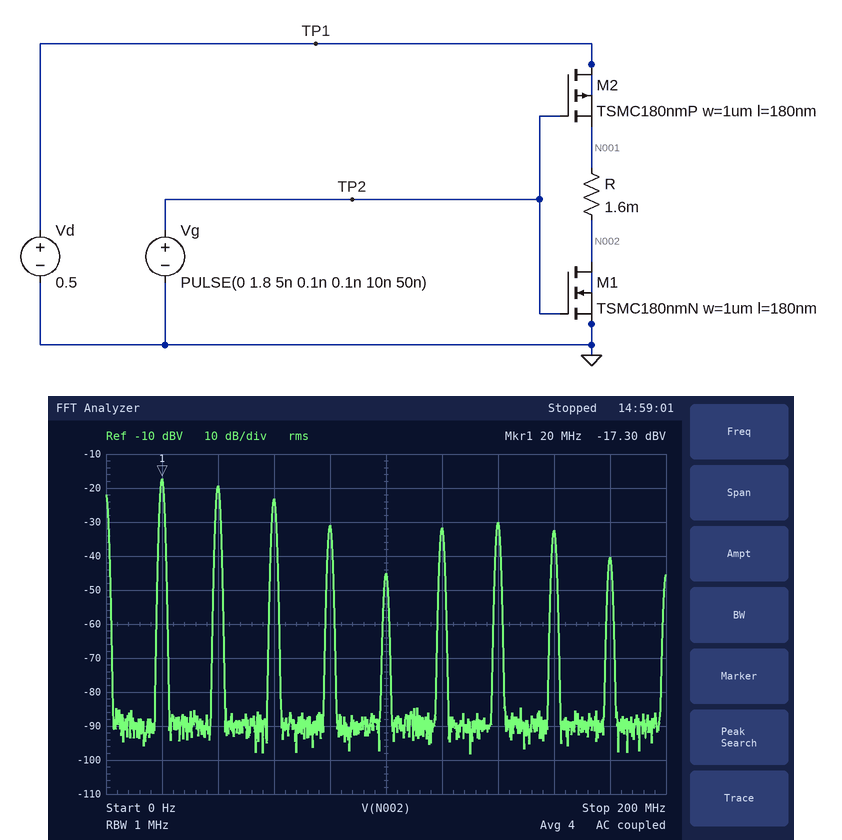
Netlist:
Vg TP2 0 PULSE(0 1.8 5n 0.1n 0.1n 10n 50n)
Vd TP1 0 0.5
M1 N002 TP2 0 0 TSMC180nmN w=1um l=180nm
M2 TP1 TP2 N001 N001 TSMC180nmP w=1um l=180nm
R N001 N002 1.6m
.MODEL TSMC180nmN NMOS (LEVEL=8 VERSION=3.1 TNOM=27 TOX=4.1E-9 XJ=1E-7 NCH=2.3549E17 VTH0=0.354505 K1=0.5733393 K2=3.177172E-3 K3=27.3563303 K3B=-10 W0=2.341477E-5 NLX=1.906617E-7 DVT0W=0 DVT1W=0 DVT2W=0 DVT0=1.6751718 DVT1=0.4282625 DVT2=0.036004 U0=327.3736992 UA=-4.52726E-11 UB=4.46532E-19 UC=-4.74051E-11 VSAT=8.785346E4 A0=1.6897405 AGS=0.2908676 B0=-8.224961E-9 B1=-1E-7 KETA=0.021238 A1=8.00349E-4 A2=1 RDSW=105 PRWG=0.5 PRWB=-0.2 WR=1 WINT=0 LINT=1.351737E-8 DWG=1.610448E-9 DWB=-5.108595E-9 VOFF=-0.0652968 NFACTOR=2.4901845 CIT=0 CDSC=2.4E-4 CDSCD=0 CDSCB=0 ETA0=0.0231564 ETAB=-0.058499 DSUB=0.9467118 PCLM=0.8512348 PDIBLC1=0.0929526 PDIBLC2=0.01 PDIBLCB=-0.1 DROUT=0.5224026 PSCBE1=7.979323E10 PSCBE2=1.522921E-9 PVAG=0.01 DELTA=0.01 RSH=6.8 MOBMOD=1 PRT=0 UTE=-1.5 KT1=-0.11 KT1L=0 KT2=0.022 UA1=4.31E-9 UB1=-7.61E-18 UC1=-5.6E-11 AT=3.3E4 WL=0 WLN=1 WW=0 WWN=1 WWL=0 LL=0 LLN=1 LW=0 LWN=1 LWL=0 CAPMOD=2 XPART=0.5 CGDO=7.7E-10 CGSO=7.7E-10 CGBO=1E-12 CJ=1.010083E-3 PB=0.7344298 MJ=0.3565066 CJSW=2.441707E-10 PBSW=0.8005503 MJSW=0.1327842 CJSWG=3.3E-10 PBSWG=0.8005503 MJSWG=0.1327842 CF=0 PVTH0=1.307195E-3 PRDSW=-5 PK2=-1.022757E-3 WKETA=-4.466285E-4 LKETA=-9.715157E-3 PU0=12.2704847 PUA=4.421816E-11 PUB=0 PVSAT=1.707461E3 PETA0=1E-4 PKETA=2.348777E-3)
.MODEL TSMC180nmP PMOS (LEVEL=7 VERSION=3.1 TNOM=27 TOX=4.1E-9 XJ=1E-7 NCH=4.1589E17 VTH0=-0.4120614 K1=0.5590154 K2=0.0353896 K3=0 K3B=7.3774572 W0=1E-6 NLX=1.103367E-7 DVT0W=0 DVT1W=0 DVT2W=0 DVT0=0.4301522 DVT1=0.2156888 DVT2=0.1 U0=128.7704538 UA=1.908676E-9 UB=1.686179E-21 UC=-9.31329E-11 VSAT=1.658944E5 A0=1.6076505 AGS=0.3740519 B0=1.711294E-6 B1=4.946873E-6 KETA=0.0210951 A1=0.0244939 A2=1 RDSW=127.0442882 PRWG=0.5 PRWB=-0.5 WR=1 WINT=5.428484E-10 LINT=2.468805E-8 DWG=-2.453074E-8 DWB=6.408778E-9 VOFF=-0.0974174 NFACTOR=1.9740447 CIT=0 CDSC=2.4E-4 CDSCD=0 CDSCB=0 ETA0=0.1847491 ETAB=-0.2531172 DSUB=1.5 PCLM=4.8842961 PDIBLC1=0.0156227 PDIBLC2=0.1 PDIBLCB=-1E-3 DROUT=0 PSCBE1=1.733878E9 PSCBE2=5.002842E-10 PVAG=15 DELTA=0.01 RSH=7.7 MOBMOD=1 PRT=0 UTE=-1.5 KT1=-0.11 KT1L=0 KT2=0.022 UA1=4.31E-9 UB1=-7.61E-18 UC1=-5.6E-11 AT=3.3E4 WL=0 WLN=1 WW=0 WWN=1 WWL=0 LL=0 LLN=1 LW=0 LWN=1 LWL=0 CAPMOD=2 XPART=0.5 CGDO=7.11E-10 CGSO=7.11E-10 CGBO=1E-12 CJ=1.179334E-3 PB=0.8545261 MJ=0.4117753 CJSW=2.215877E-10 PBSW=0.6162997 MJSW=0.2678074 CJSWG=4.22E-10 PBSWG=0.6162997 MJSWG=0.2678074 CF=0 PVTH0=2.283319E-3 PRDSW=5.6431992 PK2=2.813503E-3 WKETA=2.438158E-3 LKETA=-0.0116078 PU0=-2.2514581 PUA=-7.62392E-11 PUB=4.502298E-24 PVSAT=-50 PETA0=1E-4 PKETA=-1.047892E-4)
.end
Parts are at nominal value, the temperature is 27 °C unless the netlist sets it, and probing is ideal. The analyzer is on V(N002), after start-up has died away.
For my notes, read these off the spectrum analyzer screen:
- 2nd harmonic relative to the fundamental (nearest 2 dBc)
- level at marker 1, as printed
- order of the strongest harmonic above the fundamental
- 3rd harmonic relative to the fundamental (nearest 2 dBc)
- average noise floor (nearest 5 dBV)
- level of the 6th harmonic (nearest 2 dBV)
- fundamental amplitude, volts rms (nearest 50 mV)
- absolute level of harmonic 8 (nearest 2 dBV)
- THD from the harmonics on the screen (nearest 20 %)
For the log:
-2 dBc
-17.30 dBV
2
-6 dBc
-90 dBV
-32 dBV
150 mV
-32 dBV
100 %
